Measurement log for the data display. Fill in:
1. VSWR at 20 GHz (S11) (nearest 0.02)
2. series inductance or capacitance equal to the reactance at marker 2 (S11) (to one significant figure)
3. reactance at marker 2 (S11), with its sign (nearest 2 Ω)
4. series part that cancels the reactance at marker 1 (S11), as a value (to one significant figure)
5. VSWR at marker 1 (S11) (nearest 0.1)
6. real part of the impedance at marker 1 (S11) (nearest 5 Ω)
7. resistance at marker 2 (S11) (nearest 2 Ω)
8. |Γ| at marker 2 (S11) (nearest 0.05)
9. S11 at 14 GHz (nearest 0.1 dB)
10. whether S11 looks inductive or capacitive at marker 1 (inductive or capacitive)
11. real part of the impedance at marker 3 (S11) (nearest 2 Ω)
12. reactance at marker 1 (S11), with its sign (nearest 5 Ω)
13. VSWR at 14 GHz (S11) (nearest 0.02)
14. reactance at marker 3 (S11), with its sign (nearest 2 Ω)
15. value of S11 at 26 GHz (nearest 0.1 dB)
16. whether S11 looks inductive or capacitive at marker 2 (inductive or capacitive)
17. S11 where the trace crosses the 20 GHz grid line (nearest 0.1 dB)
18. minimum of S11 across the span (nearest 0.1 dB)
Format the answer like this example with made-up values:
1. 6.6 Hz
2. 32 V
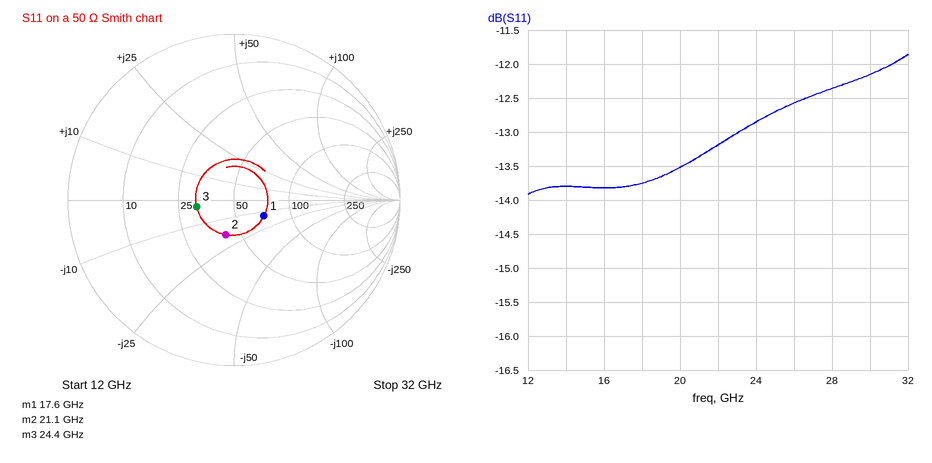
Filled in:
1. 1.54
2. 400 fF
3. -18 Ω
4. 100 pH
5. 1.5
6. 70 Ω
7. 42 Ω
8. 0.20
9. -13.8 dB
10. capacitive
11. 32 Ω
12. -15 Ω
13. 1.52
14. -2 Ω
15. -12.6 dB
16. capacitive
17. -13.5 dB
18. -13.9 dB
